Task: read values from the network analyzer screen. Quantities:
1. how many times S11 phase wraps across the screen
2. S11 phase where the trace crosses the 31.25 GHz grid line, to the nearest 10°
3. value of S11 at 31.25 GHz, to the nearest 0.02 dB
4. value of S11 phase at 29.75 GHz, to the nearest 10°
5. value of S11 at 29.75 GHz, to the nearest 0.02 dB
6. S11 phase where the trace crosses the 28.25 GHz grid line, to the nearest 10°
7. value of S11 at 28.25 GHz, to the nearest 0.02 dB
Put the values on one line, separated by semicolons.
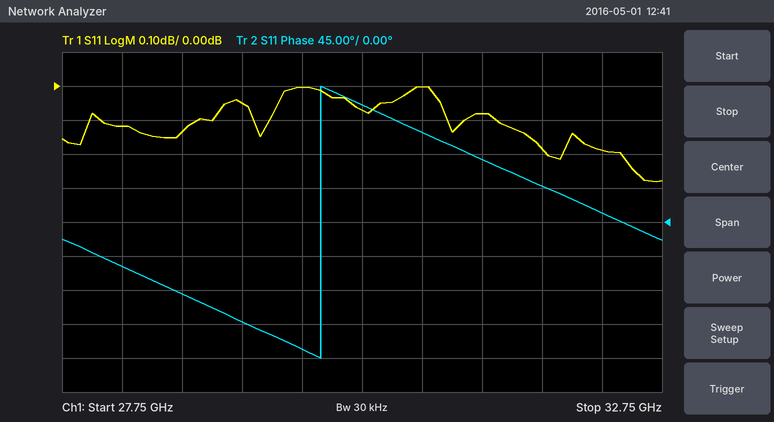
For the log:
1; 80°; -0.08 dB; -170°; 0.00 dB; -60°; -0.12 dB
